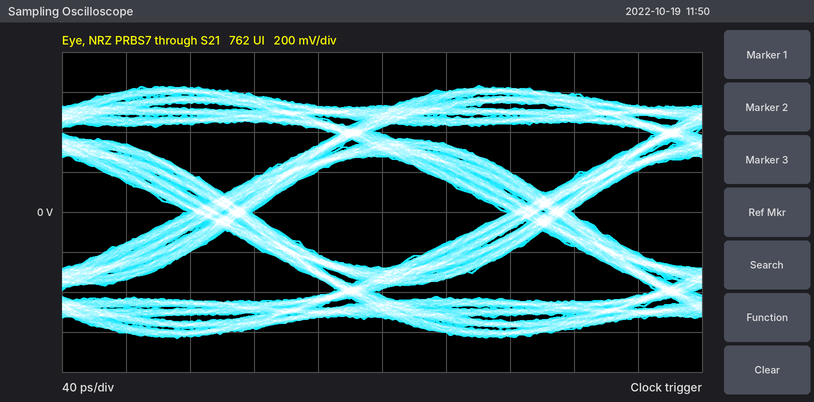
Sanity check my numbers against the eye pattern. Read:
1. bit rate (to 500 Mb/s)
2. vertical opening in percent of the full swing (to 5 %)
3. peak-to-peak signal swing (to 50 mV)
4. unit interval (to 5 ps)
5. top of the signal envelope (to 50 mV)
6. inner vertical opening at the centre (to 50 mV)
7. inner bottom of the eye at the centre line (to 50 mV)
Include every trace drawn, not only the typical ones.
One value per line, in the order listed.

5.0 Gb/s
45 %
1.25 V
200 ps
650 mV
550 mV
-300 mV
